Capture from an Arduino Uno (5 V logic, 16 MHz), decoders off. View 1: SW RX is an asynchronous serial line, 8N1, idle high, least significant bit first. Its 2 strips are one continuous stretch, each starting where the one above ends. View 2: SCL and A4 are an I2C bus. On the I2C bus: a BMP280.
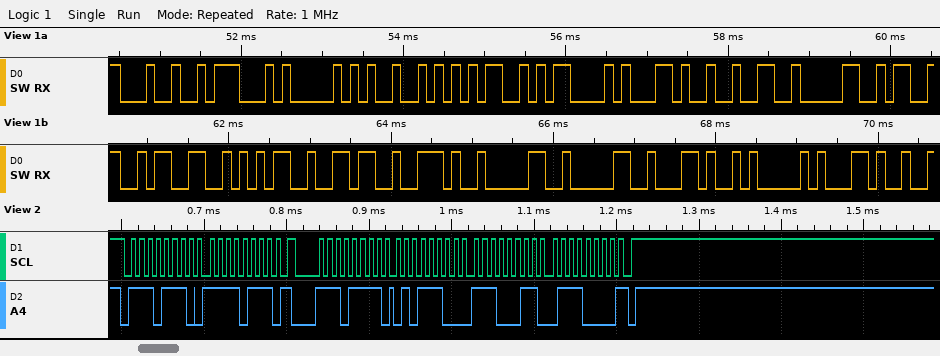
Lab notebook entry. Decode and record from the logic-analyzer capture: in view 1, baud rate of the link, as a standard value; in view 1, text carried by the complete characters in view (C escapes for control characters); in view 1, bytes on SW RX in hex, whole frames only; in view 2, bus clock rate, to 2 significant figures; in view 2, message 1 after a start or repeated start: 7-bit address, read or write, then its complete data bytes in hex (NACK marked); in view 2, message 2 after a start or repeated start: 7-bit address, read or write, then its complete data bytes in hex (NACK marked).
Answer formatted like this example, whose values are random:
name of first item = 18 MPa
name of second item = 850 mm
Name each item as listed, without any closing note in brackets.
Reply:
in view 1, baud rate of the link, as a standard value = 9600 baud
in view 1, text carried by the complete characters in view = "$GPRMC,203356.00,A,"
in view 1, bytes on SW RX in hex, whole frames only = 24 47 50 52 4D 43 2C 32 30 33 33 35 36 2E 30 30 2C 41 2C
in view 2, bus clock rate, to 2 significant figures = 100 kHz
in view 2, message 1 after a start or repeated start: 7-bit address, read or write, then its complete data bytes in hex = 0x77 write: F7
in view 2, message 2 after a start or repeated start: 7-bit address, read or write, then its complete data bytes in hex = 0x77 read: 5C E3 70 NACK
